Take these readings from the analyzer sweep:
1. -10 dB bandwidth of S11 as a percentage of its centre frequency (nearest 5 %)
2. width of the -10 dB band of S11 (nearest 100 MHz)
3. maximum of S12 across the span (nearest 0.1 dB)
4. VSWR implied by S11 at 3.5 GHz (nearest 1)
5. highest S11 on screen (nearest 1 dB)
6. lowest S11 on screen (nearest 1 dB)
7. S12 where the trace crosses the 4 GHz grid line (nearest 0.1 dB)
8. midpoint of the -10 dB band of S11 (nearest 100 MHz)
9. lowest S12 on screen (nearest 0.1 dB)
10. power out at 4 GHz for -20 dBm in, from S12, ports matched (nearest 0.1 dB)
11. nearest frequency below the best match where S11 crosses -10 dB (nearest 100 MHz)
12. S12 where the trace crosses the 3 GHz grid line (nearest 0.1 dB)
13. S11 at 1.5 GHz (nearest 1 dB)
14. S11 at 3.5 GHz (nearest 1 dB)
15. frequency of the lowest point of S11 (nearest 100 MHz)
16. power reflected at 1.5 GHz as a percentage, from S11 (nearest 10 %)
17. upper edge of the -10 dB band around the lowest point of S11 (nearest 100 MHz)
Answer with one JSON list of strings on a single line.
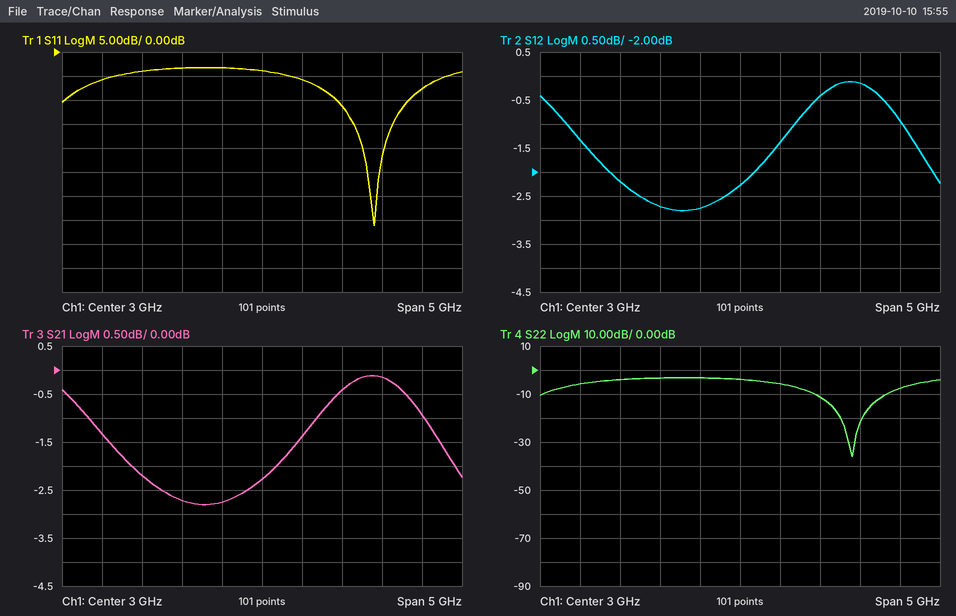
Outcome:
["20 %", "900 MHz", "-0.1 dB", "3", "-3 dB", "-36 dB", "-0.4 dB", "4.4 GHz", "-2.8 dB", "-20.4 dBm", "3.9 GHz", "-2.3 dB", "-4 dB", "-6 dB", "4.4 GHz", "40 %", "4.8 GHz"]
